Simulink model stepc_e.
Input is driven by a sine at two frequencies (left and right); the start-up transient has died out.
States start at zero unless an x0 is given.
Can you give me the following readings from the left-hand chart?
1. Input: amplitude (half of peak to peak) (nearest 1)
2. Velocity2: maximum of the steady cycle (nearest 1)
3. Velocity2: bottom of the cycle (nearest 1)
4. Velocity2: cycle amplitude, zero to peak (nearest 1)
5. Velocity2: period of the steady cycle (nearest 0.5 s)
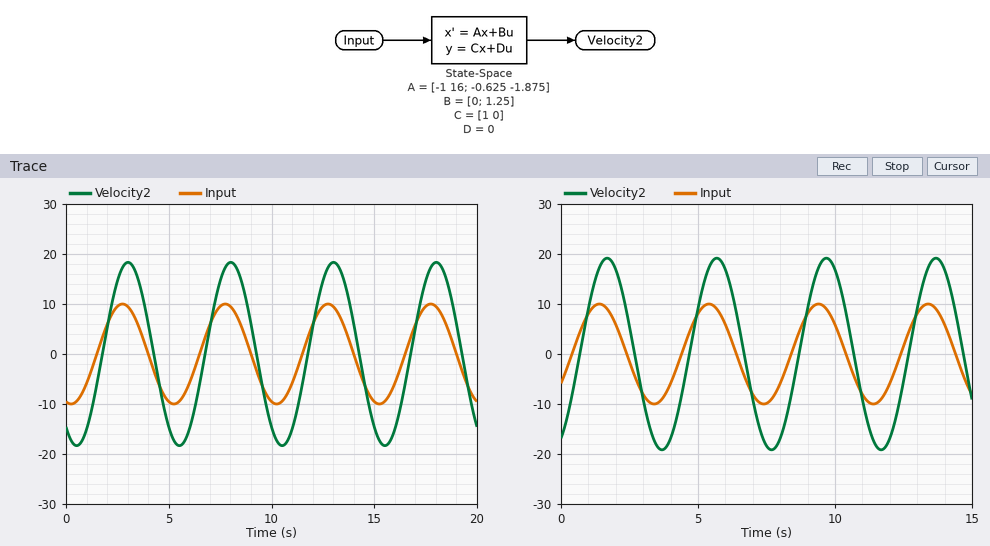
10
18
-18
18
5.0 s
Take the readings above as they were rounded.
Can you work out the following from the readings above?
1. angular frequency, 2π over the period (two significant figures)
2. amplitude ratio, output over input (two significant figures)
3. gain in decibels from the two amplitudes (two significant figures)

1.3 rad/s
1.8
5.1 dB
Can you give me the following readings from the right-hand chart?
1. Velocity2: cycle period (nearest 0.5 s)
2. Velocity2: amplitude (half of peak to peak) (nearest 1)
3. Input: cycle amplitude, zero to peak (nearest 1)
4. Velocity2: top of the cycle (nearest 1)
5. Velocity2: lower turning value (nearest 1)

4.0 s
19
10
19
-19
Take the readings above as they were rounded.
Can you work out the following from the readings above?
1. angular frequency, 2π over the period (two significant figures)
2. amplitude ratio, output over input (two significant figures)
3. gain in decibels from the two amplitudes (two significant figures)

1.6 rad/s
1.9
5.6 dB
